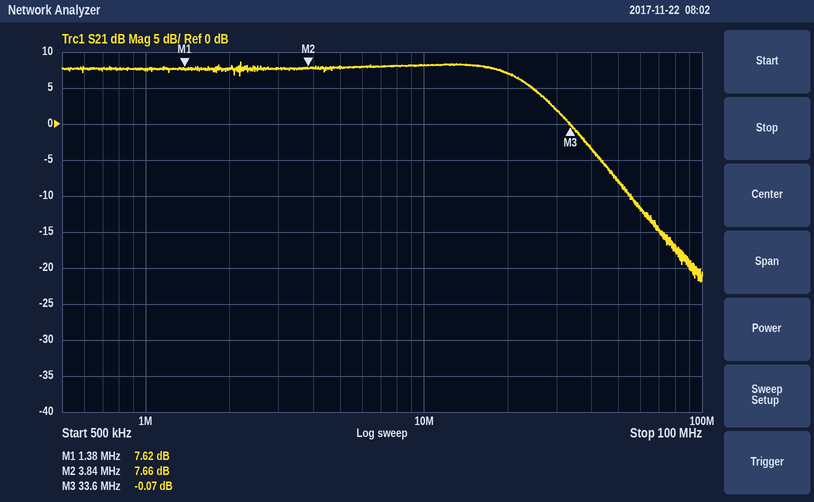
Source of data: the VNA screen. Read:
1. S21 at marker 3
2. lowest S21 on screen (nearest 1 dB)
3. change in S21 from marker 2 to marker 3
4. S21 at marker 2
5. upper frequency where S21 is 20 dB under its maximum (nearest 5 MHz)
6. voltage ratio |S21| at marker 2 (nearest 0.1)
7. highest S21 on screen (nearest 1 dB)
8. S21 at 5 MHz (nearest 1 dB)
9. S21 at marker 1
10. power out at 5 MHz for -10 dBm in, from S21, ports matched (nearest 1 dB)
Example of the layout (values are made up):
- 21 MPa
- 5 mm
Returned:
- -0.07 dB
- -22 dB
- -7.73 dB
- 7.66 dB
- 60 MHz
- 2.4
- 9 dB
- 8 dB
- 7.62 dB
- -2 dBm
